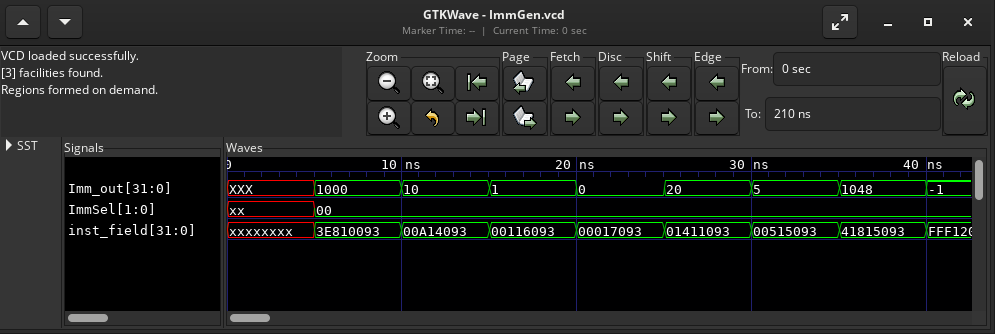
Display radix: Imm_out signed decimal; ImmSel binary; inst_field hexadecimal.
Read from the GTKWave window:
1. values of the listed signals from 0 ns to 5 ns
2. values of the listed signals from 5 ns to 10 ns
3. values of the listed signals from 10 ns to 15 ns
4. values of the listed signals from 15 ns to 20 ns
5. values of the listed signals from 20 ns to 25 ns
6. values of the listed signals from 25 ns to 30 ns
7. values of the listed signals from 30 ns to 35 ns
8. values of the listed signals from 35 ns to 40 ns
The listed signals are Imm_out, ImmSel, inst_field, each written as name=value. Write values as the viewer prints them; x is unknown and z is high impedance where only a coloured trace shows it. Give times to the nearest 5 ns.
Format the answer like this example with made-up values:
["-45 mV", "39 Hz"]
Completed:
["Imm_out=XXX, ImmSel=xx, inst_field=xxxxxxxx", "Imm_out=1000, ImmSel=00, inst_field=3E810093", "Imm_out=10, ImmSel=00, inst_field=00A14093", "Imm_out=1, ImmSel=00, inst_field=00116093", "Imm_out=0, ImmSel=00, inst_field=00017093", "Imm_out=20, ImmSel=00, inst_field=01411093", "Imm_out=5, ImmSel=00, inst_field=00515093", "Imm_out=1048, ImmSel=00, inst_field=41815093"]
